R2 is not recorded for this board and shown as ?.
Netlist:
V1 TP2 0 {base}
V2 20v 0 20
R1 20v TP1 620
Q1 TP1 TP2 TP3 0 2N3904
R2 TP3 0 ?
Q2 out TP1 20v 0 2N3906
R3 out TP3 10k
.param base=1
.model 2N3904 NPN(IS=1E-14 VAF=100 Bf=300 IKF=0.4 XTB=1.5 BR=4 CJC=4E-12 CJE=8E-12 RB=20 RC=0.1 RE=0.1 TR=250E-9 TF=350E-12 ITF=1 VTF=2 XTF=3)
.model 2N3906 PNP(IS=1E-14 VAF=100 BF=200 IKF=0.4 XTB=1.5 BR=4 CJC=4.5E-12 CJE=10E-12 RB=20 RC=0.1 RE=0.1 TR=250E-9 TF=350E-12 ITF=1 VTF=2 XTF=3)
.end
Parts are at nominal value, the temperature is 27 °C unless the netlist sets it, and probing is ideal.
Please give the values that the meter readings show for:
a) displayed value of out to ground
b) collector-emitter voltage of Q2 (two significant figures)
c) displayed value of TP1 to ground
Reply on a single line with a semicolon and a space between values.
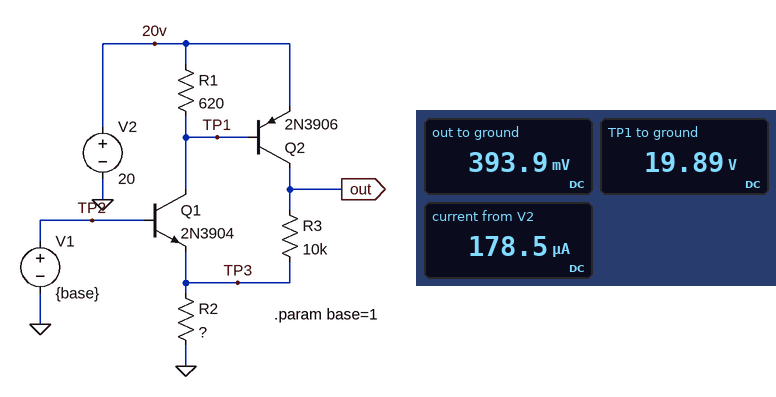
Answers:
393.9 mV; -20 V; 19.89 V
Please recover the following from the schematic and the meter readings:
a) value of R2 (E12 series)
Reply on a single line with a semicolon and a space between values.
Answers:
2.2 kΩ
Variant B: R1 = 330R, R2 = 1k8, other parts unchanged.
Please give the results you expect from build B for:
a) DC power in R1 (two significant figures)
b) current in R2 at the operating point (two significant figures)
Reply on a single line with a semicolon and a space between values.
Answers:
15 µW; 220 µA
